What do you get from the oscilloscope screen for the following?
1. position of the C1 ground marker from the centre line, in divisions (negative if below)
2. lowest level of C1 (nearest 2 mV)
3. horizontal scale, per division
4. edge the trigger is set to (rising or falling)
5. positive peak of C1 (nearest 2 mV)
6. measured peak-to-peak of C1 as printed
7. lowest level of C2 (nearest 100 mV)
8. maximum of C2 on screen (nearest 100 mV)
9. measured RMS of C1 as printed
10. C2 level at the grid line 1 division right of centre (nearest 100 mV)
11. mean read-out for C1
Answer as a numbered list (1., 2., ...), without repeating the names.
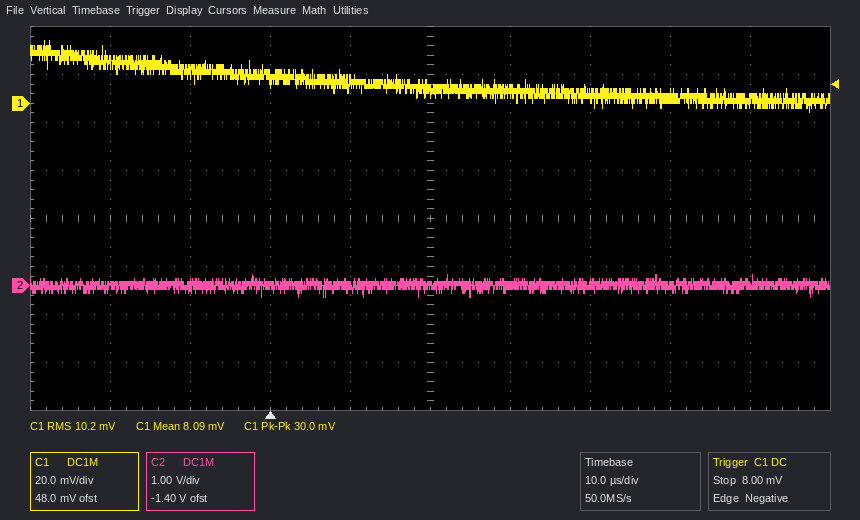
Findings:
1. +2.4 div
2. -4 mV
3. 10 µs
4. falling
5. 26 mV
6. 30.0 mV
7. -200 mV
8. 200 mV
9. 10.2 mV
10. 0.0 V
11. 8.09 mV
